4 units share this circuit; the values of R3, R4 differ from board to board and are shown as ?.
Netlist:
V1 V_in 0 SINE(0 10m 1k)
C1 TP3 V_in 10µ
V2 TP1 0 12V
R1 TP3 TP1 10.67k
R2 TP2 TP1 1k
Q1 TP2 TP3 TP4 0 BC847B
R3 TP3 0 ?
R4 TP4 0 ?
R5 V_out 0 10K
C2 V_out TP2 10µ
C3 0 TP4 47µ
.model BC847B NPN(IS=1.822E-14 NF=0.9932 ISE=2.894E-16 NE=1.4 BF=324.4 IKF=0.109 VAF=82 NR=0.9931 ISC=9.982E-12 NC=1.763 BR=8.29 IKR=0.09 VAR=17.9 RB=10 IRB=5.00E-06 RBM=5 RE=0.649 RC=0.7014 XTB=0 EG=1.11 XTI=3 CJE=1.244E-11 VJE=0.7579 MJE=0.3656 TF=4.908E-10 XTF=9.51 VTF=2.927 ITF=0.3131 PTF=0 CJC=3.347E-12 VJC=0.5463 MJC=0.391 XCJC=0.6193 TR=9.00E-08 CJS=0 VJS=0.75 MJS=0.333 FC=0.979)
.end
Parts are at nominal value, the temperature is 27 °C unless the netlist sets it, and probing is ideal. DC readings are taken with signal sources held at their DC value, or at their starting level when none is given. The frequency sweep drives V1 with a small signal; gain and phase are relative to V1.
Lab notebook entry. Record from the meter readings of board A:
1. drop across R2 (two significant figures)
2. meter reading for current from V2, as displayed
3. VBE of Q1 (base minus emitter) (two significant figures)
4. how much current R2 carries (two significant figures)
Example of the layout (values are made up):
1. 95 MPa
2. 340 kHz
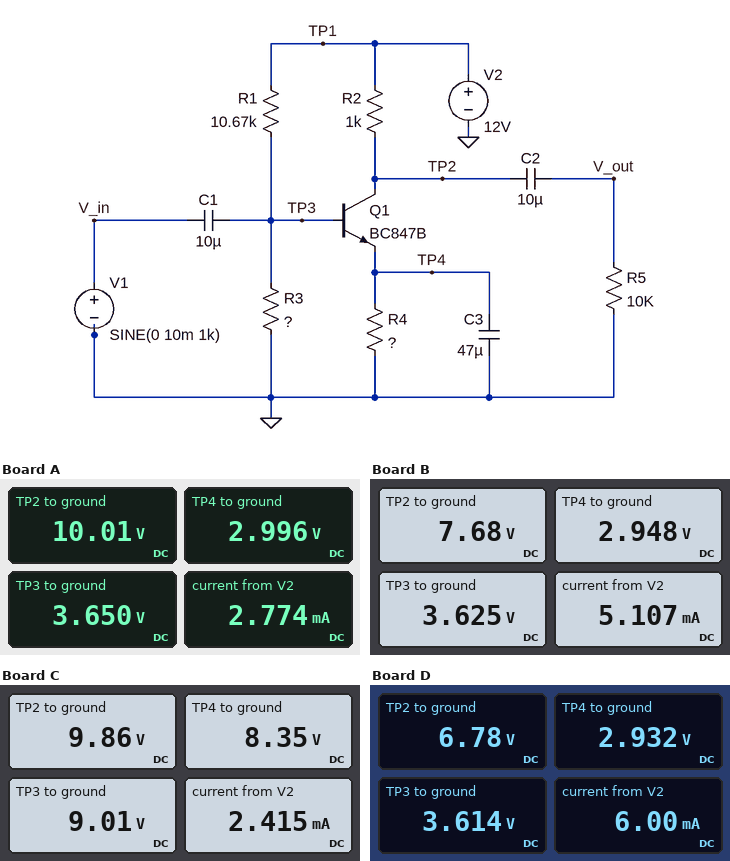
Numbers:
1. 2.0 V
2. 2.774 mA
3. 650 mV
4. 2.0 mA
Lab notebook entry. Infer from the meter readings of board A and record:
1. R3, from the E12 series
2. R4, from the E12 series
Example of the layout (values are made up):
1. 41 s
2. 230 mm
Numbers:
1. 4.7 kΩ
2. 1.5 kΩ
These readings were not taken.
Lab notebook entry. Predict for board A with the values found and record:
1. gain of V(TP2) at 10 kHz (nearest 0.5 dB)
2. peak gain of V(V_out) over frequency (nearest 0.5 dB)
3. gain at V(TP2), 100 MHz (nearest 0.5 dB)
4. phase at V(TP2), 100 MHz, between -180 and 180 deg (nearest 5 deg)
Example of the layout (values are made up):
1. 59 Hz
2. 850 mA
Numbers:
1. 36.0 dB
2. 36.0 dB
3. 33.0 dB
4. 120 deg
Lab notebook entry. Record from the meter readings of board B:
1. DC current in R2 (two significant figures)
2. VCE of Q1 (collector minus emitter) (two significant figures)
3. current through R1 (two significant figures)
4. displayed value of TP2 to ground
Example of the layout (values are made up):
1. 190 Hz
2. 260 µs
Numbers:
1. 4.3 mA
2. 4.7 V
3. 780 µA
4. 7.68 V
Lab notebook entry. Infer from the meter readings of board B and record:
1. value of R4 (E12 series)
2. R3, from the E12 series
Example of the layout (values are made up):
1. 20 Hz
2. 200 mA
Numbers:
1. 680 Ω
2. 4.7 kΩ
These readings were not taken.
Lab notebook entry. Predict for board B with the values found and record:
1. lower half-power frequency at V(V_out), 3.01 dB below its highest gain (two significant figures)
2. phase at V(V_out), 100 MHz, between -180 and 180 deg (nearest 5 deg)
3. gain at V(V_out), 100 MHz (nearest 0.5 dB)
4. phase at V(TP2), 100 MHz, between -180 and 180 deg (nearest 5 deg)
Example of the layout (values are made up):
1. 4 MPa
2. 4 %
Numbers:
1. 490 Hz
2. 110 deg
3. 37.0 dB
4. 110 deg
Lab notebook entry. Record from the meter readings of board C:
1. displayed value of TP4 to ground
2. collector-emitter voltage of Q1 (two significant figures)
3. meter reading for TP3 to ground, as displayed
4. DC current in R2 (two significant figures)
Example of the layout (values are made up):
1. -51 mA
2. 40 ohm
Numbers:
1. 8.35 V
2. 1.5 V
3. 9.01 V
4. 2.1 mA
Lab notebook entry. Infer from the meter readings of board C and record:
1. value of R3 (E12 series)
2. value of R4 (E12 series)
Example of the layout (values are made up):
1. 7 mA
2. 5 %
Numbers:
1. 33 kΩ
2. 3.9 kΩ
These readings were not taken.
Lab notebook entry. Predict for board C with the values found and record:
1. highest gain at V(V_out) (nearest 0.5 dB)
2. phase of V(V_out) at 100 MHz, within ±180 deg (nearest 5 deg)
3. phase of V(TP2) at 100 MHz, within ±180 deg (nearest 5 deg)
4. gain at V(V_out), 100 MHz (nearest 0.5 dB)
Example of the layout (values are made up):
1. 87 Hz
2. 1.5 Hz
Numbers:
1. 36.5 dB
2. 105 deg
3. 105 deg
4. 30.0 dB
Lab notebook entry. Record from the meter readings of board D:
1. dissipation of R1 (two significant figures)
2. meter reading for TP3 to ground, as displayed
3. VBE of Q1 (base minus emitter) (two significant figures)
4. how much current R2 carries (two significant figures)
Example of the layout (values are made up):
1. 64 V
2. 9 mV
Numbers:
1. 6.6 mW
2. 3.614 V
3. 680 mV
4. 5.2 mA
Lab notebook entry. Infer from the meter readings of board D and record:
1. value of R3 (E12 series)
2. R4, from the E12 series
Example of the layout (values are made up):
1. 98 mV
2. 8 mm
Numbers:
1. 4.7 kΩ
2. 560 Ω
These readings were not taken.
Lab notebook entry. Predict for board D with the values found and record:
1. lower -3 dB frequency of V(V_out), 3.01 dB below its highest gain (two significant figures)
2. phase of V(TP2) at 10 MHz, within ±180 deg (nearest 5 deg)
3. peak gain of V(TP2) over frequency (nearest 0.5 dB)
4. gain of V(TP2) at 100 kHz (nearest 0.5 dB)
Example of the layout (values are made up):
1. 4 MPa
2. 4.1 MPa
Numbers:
1. 570 Hz
2. 170 deg
3. 43.5 dB
4. 43.5 dB
